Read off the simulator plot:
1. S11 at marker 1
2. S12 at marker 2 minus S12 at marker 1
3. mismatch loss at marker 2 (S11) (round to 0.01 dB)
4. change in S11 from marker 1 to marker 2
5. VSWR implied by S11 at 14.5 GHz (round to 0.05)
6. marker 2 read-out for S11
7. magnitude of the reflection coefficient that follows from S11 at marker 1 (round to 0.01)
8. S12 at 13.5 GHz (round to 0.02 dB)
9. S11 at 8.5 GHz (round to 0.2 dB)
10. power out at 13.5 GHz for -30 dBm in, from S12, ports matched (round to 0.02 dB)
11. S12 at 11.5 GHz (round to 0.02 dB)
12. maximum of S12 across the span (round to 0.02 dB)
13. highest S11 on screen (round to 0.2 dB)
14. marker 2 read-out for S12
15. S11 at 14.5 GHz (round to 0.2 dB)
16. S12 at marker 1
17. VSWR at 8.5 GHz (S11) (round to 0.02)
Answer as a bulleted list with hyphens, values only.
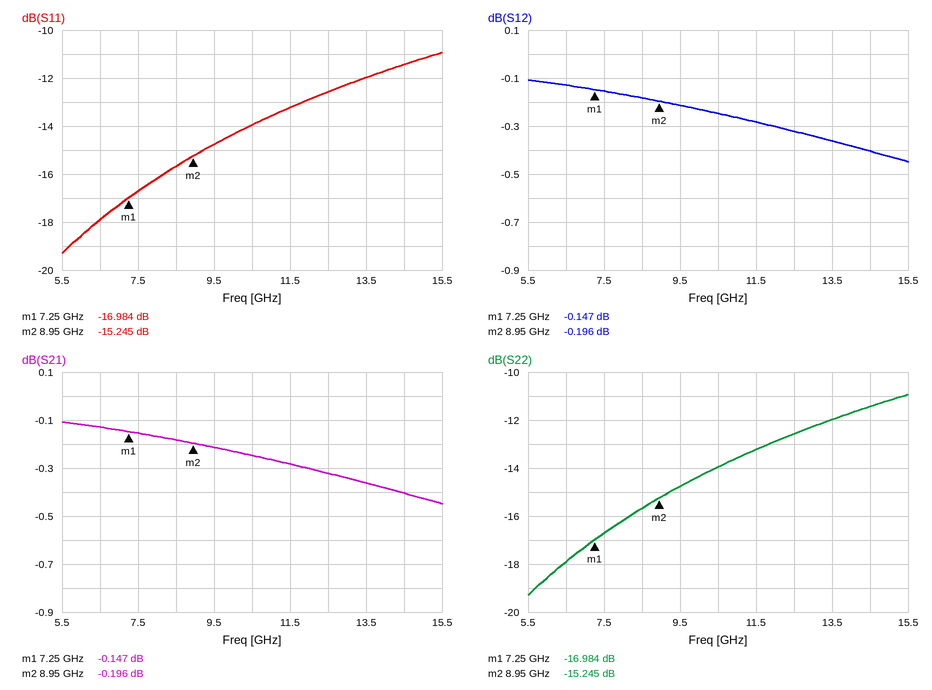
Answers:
- -16.984 dB
- -0.049 dB
- 0.13 dB
- 1.739 dB
- 1.75
- -15.245 dB
- 0.14
- -0.36 dB
- -15.6 dB
- -30.36 dBm
- -0.28 dB
- -0.10 dB
- -11.0 dB
- -0.196 dB
- -11.4 dB
- -0.147 dB
- 1.40
